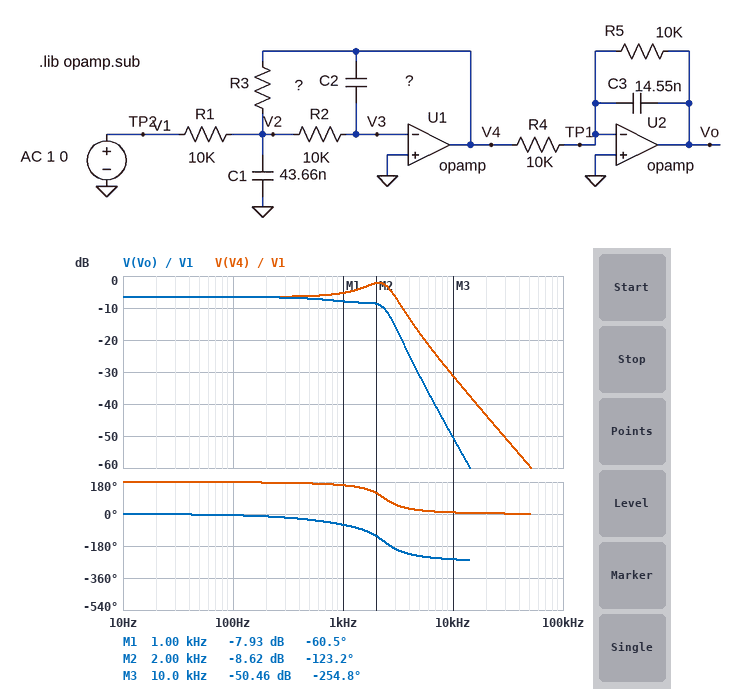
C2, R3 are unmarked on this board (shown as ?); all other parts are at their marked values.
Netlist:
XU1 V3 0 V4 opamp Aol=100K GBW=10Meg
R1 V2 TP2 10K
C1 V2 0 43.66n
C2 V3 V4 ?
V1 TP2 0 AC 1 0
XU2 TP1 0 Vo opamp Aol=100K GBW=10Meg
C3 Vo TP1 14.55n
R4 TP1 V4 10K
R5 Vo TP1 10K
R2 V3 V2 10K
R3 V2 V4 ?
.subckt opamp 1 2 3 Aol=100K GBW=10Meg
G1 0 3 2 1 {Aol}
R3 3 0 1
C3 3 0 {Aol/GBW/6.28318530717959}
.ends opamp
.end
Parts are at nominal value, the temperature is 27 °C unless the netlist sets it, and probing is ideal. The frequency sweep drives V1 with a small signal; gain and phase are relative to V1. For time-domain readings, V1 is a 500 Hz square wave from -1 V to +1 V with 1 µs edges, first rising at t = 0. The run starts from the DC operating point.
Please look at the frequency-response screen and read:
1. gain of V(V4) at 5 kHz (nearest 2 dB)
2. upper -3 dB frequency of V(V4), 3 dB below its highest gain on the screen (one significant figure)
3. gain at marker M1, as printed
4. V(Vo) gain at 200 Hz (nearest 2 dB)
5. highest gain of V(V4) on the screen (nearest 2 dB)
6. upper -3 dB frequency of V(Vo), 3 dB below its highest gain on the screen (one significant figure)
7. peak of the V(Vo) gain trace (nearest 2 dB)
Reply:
-18 dB
3 kHz
-7.93 dB
-6 dB
-2 dB
2 kHz
-6 dB
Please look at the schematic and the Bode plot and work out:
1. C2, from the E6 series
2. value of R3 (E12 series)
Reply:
2.2 nF
4.7 kΩ
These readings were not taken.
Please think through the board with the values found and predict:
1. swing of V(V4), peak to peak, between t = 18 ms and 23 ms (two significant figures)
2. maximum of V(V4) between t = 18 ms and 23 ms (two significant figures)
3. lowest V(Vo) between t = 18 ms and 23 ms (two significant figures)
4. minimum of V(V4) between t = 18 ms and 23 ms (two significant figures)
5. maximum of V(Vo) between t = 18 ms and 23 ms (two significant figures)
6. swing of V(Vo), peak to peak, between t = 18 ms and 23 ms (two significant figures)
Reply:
1.6 V
800 mV
-480 mV
-800 mV
480 mV
950 mV
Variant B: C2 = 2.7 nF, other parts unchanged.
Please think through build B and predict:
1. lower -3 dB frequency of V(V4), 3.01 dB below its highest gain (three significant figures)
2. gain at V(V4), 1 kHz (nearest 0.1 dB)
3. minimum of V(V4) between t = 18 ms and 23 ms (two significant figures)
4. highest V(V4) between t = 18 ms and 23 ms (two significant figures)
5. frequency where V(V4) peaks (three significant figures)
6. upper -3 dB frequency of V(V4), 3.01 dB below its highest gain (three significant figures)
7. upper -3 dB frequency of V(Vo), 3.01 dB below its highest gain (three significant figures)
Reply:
655 Hz
-5.1 dB
-760 mV
760 mV
1.85 kHz
2.54 kHz
2.02 kHz
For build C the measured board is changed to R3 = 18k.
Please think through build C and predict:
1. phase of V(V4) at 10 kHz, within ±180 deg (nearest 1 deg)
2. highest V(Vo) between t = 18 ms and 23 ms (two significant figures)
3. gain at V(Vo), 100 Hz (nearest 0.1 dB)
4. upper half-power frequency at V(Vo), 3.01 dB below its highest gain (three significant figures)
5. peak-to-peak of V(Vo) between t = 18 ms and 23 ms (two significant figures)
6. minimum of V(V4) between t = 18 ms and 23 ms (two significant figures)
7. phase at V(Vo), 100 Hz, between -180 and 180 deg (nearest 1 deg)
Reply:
5 deg
2.3 V
5.1 dB
1.31 kHz
4.5 V
-2.7 V
-9 deg
